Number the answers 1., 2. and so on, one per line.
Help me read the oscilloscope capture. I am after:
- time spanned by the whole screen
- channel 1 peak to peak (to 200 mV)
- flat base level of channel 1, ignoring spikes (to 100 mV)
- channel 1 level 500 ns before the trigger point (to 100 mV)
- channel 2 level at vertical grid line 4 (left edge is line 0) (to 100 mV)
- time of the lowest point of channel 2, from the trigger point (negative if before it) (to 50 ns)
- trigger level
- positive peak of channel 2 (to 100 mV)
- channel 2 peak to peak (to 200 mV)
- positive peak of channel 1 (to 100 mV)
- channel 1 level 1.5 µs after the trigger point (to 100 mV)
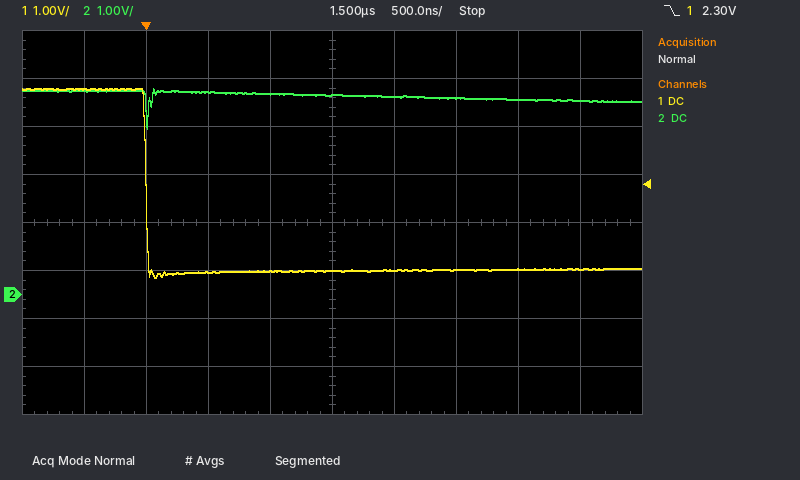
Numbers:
1. 5 µs
2. 4.0 V
3. 500 mV
4. 4.3 V
5. 4.2 V
6. 0 ns
7. 2.30 V
8. 4.3 V
9. 800 mV
10. 4.3 V
11. 500 mV
